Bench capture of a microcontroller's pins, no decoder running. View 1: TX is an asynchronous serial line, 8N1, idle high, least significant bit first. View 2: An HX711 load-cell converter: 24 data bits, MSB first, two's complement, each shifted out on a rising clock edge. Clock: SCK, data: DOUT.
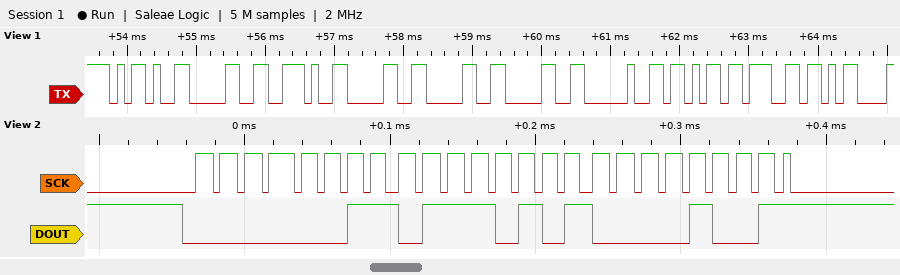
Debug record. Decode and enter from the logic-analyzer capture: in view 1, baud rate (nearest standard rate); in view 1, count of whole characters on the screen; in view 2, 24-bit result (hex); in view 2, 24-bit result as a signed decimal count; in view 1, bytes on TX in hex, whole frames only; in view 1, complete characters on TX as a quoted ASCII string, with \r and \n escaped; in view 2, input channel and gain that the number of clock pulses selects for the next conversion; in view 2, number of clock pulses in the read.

9600 baud
10
0x037509
226569
2D 30 2E 30 30 30 20 6B 67 0D
"-0.000 kg\r"
channel A, gain 128
25
